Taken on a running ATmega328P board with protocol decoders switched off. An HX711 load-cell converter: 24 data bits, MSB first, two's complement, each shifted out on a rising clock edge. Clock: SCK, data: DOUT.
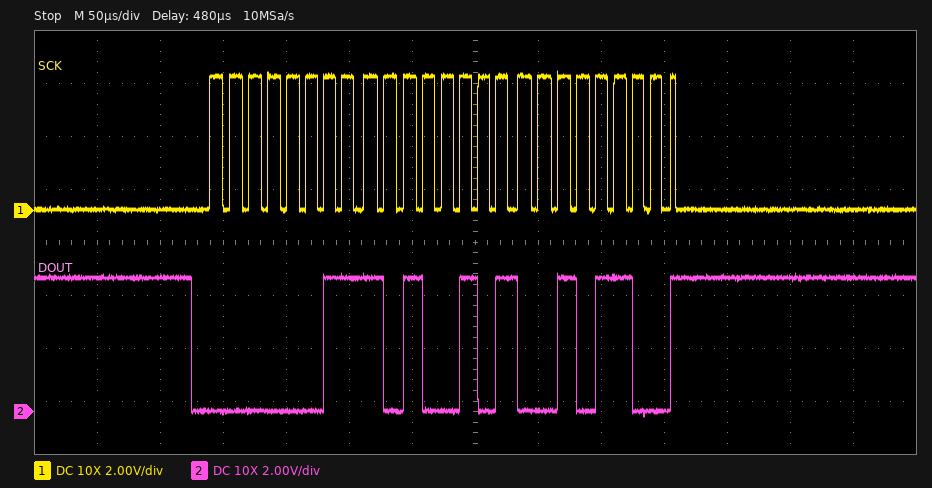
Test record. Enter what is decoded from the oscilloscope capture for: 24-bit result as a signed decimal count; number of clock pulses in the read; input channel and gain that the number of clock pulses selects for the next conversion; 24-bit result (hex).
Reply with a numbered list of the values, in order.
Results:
1. 238892
2. 25
3. channel A, gain 128
4. 0x03A52C
